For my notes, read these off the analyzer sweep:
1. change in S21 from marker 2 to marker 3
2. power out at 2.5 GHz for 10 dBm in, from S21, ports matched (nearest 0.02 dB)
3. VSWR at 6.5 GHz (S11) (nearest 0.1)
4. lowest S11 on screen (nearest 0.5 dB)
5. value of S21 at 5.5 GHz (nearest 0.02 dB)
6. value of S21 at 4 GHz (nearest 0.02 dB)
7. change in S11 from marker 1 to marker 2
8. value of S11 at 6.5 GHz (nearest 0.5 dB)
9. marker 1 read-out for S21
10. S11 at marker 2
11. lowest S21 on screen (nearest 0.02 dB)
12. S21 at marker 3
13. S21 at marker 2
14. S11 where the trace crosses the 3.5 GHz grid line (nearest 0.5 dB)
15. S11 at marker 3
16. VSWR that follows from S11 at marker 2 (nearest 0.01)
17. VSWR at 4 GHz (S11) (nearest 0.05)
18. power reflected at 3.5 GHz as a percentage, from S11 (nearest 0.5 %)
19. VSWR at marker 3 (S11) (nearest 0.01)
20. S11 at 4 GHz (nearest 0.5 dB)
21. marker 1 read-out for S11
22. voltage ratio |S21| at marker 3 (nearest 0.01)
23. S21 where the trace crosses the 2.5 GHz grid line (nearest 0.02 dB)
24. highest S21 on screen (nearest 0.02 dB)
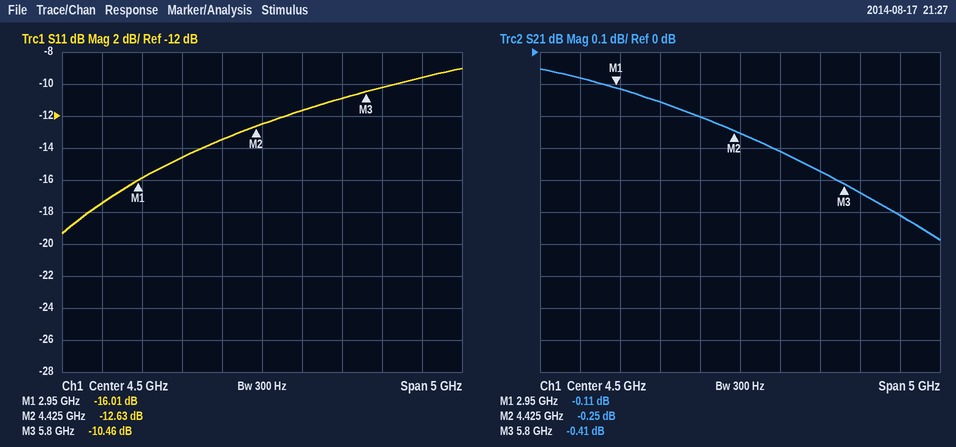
-0.16 dB
9.92 dBm
2.0
-19.5 dB
-0.38 dB
-0.20 dB
3.38 dB
-9.5 dB
-0.11 dB
-12.63 dB
-0.58 dB
-0.41 dB
-0.25 dB
-14.5 dB
-10.46 dB
1.61
1.55
3.5 %
1.86
-13.5 dB
-16.01 dB
0.95
-0.08 dB
-0.06 dB
